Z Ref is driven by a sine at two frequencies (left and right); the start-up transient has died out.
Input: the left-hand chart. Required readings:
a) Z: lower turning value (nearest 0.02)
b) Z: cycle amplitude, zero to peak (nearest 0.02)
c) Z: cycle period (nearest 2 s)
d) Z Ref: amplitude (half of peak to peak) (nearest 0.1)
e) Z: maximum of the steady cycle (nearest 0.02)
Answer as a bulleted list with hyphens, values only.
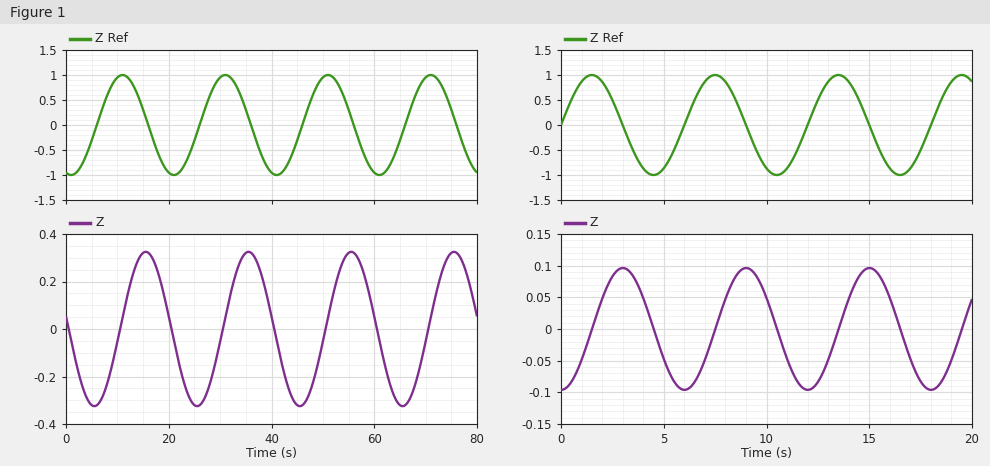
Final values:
- -0.32
- 0.32
- 20 s
- 1.0
- 0.32
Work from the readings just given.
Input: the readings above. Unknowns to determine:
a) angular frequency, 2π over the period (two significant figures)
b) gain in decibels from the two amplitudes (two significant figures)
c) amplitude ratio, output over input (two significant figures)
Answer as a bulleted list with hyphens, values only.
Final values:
- 0.31 rad/s
- -9.9 dB
- 0.32
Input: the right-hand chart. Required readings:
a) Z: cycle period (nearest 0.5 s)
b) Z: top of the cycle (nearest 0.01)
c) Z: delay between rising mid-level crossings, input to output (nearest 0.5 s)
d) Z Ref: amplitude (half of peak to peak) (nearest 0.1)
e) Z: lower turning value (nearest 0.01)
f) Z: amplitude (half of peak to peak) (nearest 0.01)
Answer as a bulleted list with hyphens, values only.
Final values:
- 6.0 s
- 0.10
- 1.5 s
- 1.0
- -0.10
- 0.10
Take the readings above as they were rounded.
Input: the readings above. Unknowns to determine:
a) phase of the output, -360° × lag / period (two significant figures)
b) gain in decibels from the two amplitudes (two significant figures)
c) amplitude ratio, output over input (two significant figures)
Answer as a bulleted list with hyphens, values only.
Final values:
- -90°
- -20 dB
- 0.10
